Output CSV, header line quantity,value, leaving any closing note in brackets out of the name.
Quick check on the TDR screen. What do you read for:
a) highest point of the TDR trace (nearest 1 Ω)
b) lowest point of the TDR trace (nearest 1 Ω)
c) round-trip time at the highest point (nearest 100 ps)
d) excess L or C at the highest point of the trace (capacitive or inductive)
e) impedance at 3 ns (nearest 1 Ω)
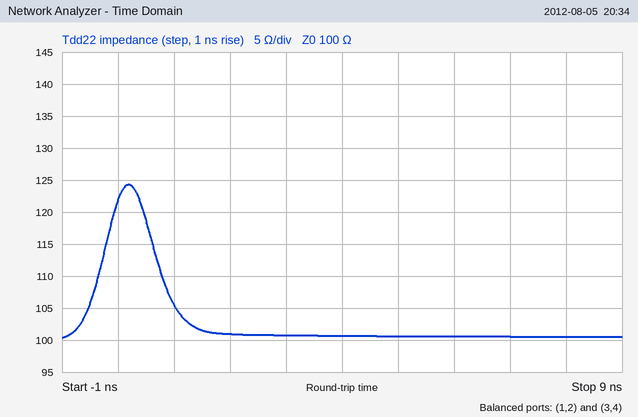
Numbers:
quantity,value
highest point of the TDR trace,124 Ω
lowest point of the TDR trace,100 Ω
round-trip time at the highest point,200 ps
excess L or C at the highest point of the trace,inductive
impedance at 3 ns,101 Ω
